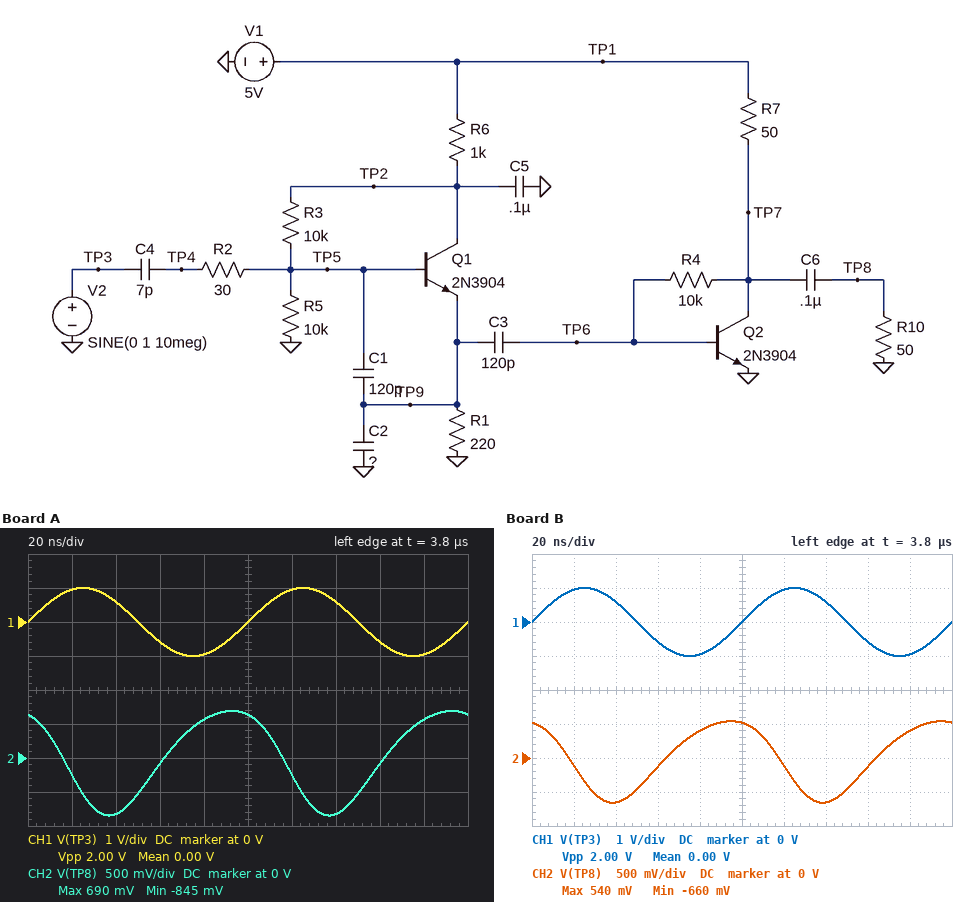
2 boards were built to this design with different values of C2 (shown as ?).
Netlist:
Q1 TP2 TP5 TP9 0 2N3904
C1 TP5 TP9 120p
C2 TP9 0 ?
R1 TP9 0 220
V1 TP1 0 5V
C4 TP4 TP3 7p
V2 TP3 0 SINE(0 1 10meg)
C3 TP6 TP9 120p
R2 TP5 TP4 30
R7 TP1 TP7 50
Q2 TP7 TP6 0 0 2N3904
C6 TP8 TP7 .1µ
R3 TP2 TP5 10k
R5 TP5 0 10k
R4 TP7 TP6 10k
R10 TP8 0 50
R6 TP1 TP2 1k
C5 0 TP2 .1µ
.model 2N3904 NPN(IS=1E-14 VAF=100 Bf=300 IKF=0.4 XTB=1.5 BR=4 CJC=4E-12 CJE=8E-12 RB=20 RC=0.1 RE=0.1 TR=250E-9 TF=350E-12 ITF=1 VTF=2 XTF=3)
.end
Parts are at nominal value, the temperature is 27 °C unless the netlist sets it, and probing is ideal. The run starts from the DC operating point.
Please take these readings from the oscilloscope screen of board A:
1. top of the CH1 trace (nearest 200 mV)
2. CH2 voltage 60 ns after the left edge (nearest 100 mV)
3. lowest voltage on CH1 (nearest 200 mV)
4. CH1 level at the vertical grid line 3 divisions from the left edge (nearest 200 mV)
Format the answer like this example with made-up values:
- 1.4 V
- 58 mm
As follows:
- 1.0 V
- -100 mV
- -1.0 V
- -600 mV
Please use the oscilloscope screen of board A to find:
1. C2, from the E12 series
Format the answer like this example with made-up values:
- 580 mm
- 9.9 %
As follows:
- 220 pF
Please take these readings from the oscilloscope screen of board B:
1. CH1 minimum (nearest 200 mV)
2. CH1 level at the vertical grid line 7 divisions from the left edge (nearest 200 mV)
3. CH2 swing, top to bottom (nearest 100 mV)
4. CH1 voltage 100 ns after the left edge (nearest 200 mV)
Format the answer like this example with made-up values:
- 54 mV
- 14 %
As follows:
- -1.0 V
- 600 mV
- 1.2 V
- 0 V
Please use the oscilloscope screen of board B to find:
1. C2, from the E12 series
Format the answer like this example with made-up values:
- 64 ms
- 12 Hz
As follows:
- 330 pF
